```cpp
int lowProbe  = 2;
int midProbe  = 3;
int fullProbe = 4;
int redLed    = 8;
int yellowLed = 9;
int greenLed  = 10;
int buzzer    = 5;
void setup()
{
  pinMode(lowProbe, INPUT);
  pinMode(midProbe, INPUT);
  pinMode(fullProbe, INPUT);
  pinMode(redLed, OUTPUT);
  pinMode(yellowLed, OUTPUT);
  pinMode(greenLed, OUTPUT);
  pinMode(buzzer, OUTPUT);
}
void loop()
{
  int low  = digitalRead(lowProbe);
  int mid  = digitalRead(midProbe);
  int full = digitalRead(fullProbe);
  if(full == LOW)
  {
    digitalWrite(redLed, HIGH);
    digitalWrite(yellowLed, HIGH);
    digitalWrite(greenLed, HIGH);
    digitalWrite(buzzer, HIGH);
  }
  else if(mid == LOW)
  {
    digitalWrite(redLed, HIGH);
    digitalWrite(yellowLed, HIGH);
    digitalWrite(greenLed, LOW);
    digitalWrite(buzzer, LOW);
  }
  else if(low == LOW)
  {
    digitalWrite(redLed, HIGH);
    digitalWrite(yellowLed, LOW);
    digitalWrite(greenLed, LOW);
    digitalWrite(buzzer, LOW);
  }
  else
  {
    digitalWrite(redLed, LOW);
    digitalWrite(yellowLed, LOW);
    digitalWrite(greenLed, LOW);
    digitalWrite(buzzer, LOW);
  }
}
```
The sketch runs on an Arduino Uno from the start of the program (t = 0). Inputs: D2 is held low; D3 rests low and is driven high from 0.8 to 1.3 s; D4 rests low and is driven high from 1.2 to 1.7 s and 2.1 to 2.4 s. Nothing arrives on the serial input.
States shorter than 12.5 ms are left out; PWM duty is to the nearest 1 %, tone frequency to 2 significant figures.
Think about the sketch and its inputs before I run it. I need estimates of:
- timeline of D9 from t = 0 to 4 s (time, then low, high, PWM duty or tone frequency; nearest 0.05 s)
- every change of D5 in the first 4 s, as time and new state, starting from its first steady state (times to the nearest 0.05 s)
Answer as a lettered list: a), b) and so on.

a) 0 s high; 1.2 s low; 1.3 s high
b) 0 s high; 1.2 s low; 1.7 s high; 2.1 s low; 2.4 s high
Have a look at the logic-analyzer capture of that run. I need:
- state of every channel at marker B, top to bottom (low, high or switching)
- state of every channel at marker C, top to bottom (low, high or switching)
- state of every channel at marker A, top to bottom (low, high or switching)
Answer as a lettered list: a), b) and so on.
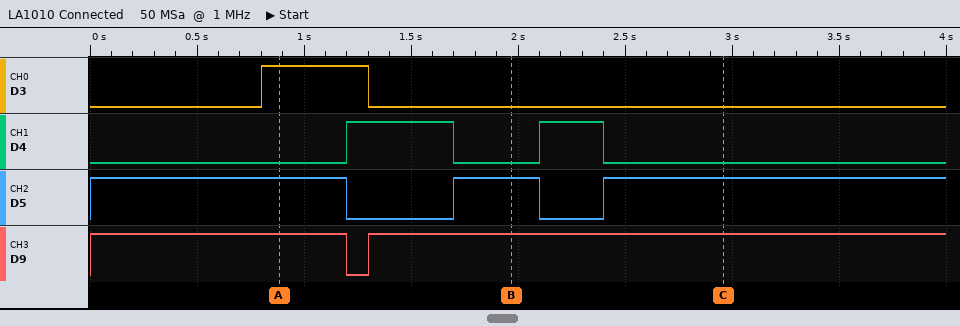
a) D3 low, D4 low, D5 high, D9 high
b) D3 low, D4 low, D5 high, D9 high
c) D3 high, D4 low, D5 high, D9 high
